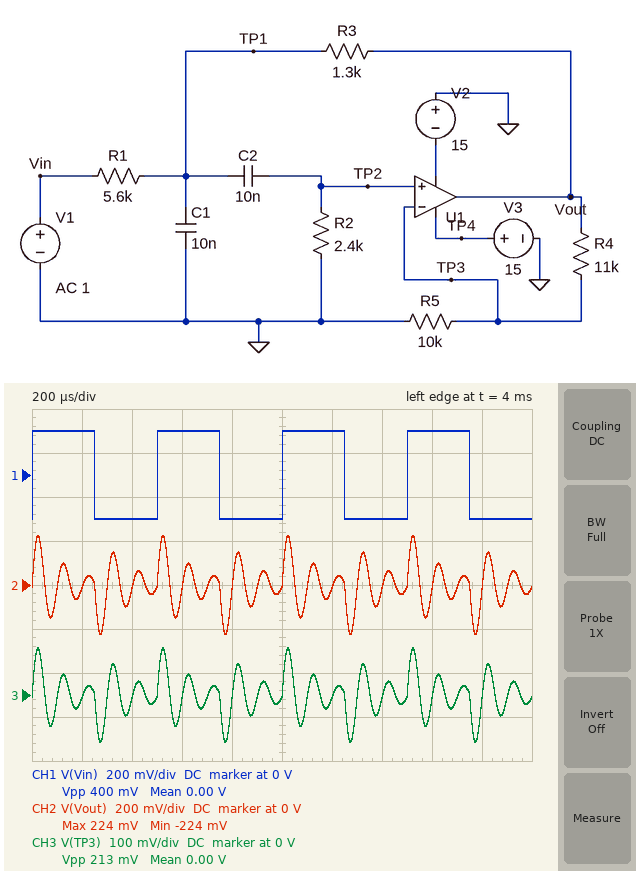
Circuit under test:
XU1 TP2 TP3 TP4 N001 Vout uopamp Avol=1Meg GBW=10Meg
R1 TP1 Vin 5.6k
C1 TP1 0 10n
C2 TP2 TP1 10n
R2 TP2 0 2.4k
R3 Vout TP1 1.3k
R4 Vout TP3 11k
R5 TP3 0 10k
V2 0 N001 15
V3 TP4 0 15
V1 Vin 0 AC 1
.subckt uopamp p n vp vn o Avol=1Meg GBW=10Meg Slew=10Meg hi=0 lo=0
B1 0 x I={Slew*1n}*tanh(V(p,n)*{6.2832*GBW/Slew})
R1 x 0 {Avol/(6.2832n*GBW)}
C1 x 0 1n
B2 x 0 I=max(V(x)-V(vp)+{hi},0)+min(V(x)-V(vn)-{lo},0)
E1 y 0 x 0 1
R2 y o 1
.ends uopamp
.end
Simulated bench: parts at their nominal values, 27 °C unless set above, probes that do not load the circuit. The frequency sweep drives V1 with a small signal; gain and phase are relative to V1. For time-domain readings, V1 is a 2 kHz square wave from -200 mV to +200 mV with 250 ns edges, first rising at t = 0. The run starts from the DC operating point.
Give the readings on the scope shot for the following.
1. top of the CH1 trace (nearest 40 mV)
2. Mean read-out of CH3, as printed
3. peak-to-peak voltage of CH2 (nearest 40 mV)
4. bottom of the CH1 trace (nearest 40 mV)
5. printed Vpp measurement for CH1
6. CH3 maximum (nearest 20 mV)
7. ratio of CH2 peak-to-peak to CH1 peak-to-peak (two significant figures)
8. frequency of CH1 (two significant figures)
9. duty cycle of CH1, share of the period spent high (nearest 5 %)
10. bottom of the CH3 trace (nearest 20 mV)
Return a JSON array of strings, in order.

["200 mV", "0.00 V", "440 mV", "-200 mV", "400 mV", "100 mV", "1.1", "2.0 kHz", "50 %", "-100 mV"]
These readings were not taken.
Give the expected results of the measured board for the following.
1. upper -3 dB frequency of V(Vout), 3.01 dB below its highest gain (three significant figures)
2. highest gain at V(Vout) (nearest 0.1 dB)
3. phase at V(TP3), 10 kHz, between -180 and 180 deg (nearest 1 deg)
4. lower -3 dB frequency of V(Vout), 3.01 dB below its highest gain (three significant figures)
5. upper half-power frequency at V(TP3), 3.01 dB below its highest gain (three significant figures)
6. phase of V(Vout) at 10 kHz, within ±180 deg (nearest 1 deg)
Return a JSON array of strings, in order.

["11.4 kHz", "7.1 dB", "-1 deg", "8.75 kHz", "11.4 kHz", "-1 deg"]
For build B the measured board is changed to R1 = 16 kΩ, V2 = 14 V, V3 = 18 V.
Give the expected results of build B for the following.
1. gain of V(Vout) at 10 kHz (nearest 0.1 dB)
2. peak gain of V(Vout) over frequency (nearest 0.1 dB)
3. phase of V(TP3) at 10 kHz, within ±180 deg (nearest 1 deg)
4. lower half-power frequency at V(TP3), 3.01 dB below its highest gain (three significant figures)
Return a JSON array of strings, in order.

["2.9 dB", "8.4 dB", "-58 deg", "8.96 kHz"]
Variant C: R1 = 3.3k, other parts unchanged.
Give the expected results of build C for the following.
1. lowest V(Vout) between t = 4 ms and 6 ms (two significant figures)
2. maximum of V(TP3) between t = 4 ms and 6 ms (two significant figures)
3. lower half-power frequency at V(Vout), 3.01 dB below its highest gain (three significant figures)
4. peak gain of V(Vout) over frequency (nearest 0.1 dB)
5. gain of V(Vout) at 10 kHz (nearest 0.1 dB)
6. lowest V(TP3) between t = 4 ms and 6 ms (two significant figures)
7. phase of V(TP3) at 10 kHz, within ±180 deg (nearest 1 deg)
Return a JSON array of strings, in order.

["-290 mV", "140 mV", "8.56 kHz", "6.8 dB", "6.5 dB", "-140 mV", "15 deg"]
